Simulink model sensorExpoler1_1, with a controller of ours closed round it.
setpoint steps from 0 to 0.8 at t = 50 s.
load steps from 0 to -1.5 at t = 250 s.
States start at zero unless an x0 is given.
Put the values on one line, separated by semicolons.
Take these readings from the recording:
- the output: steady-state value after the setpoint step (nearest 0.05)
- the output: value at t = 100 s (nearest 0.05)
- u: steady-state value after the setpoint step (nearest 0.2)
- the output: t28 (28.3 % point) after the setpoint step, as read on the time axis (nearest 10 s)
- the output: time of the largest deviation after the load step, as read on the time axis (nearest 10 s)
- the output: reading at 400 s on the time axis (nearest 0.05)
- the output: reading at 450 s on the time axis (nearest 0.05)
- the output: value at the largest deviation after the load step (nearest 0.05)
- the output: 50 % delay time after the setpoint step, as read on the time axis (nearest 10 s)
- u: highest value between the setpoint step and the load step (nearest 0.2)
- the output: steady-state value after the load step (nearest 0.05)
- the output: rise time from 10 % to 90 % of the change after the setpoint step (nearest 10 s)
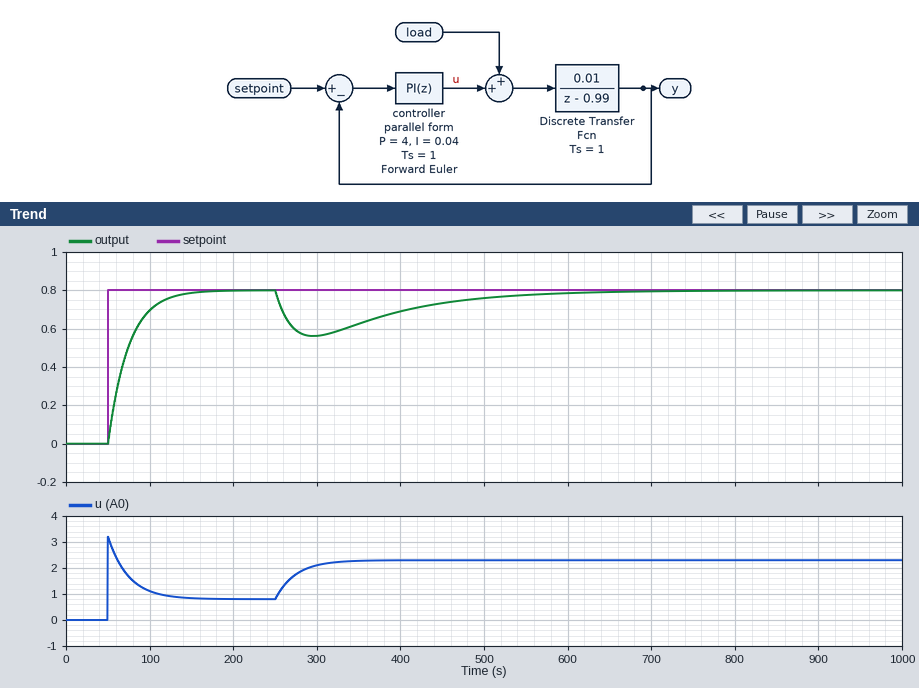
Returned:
0.80; 0.70; 0.8; 60 s; 300 s; 0.70; 0.75; 0.55; 70 s; 3.2; 0.80; 50 s
